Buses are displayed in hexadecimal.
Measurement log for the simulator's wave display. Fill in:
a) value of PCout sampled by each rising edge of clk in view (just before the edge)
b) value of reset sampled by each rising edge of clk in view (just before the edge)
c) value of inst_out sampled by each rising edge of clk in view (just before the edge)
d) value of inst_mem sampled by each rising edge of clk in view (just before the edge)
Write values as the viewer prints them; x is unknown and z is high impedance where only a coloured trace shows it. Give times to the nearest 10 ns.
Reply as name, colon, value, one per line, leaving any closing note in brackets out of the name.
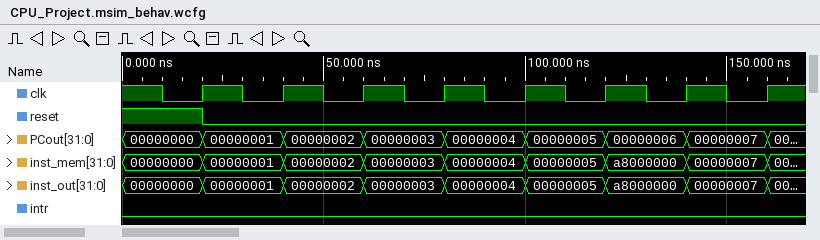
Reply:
value of PCout sampled by each rising edge of clk in view: 00000000, 00000001, 00000002, 00000003, 00000004, 00000005, 00000006, 00000007
value of reset sampled by each rising edge of clk in view: 1 0 0 0 0 0 0 0
value of inst_out sampled by each rising edge of clk in view: 00000000, 00000001, 00000002, 00000003, 00000004, 00000005, a8000000, 00000007
value of inst_mem sampled by each rising edge of clk in view: 00000000, 00000001, 00000002, 00000003, 00000004, 00000005, a8000000, 00000007
